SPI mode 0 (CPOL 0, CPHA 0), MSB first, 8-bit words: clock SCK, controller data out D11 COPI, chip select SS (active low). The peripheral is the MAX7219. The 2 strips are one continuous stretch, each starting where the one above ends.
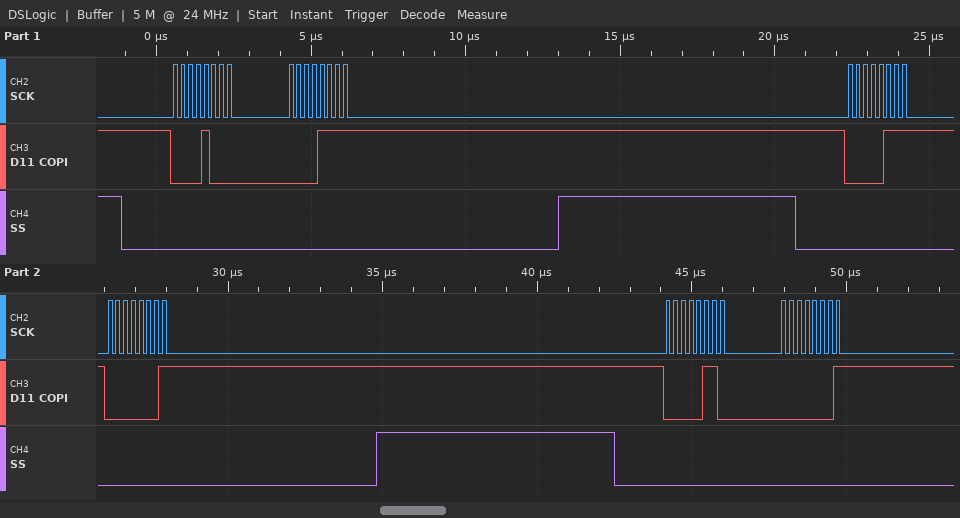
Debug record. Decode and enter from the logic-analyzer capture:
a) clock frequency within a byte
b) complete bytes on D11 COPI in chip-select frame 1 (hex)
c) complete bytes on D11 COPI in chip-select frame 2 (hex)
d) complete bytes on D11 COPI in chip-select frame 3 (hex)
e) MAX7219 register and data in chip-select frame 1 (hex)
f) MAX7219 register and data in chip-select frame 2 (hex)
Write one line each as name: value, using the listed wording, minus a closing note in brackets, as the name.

clock frequency within a byte: 4 MHz
complete bytes on D11 COPI in chip-select frame 1: 08 0F
complete bytes on D11 COPI in chip-select frame 2: 07 01
complete bytes on D11 COPI in chip-select frame 3: 06 01
MAX7219 register and data in chip-select frame 1: register 0x8, data 0x0F
MAX7219 register and data in chip-select frame 2: register 0x7, data 0x01
